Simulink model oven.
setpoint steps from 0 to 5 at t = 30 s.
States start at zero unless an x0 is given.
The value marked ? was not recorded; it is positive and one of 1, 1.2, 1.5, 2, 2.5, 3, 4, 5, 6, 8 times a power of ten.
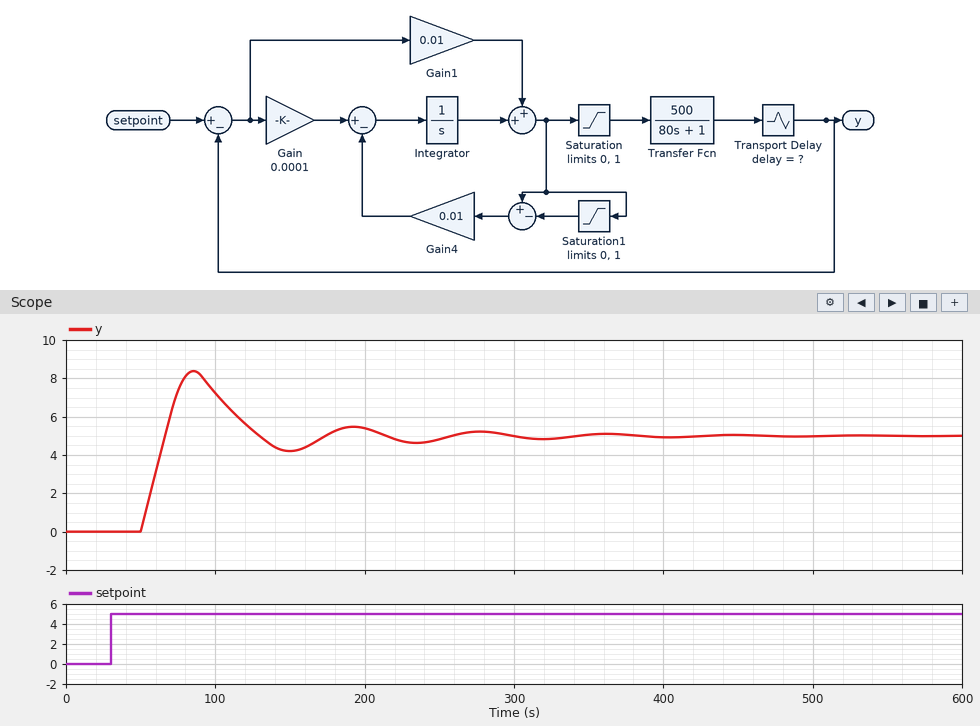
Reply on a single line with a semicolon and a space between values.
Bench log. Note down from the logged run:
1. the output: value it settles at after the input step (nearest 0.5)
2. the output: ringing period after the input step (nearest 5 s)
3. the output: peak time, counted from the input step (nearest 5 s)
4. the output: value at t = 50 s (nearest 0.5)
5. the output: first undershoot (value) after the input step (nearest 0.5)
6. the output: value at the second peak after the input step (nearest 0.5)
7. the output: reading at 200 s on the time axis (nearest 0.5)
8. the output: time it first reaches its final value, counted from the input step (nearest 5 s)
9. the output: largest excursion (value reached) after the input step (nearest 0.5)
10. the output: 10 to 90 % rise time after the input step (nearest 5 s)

5.0; 105 s; 55 s; 0.0; 4.0; 5.5; 5.5; 35 s; 8.5; 15 s
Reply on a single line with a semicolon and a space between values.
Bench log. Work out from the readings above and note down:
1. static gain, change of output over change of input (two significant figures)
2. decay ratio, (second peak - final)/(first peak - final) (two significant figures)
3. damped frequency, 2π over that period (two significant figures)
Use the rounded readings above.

1.0; 0.14; 0.060 rad/s
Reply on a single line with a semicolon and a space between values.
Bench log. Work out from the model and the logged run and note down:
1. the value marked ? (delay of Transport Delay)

20
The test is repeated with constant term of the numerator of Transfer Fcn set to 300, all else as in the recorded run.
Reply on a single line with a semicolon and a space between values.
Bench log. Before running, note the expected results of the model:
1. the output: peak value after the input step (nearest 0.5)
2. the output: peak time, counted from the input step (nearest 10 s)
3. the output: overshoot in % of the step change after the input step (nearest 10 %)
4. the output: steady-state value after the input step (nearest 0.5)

6.0; 70 s; 20 %; 5.0
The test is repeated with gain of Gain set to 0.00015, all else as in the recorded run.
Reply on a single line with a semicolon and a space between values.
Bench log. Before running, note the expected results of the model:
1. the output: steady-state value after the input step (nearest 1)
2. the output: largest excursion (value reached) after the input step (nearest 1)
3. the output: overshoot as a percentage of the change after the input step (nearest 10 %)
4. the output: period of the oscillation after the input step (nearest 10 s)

5; 9; 80 %; 120 s
